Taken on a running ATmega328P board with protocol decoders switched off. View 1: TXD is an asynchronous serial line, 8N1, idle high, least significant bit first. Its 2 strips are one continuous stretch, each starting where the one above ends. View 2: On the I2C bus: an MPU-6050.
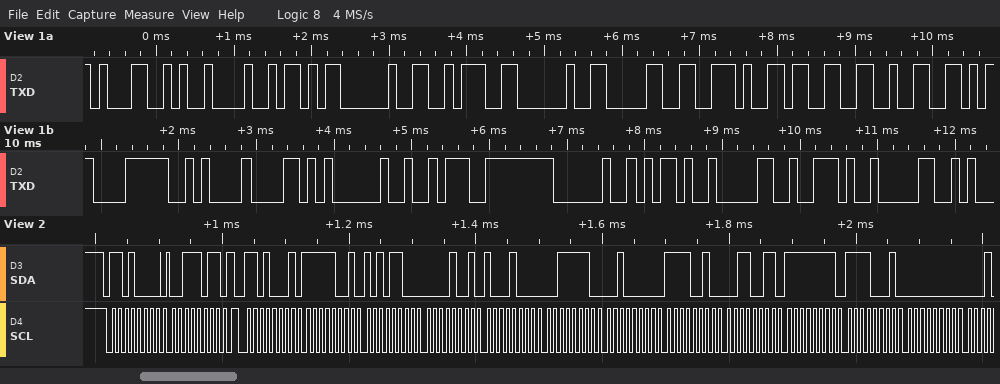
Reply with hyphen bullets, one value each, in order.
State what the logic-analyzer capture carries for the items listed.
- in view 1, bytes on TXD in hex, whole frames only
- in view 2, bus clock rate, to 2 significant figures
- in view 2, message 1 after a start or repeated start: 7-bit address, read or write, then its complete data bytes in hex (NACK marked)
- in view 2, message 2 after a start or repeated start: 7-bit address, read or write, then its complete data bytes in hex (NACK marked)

- 31 09 5A 20 3A 20 30 2E 33 32 0D 0A 58 20 3A 20 2D 30 2E 30
- 100 kHz
- 0x68 write: 3B
- 0x68 read: F9 AC 09 88 3E 20 F2 33 FF F1 00
